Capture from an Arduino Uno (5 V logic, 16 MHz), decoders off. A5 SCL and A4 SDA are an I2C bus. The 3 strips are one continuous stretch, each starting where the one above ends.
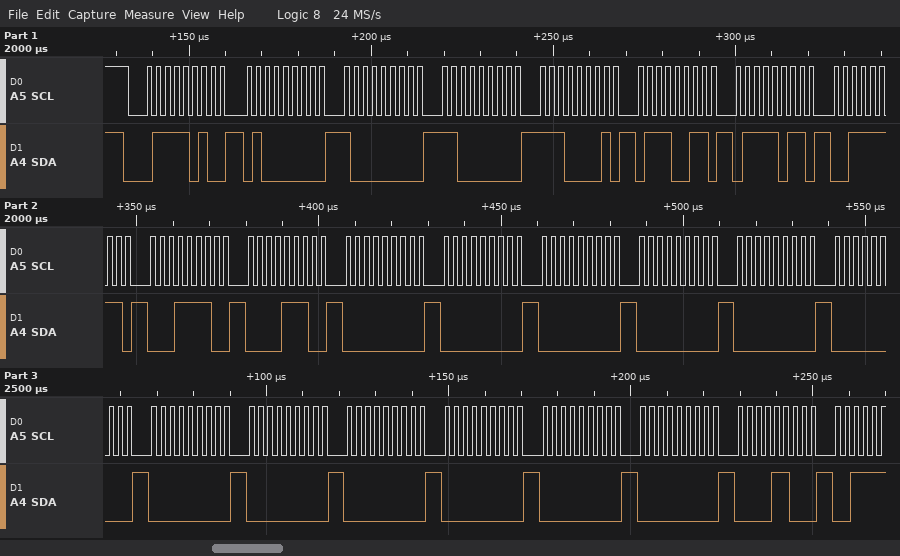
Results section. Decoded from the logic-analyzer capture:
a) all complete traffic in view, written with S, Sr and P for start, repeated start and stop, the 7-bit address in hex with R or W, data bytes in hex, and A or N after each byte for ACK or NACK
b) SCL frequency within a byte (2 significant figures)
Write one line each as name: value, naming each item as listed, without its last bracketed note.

all complete traffic in view, written with S, Sr and P for start, repeated start and stop, the 7-bit address in hex with R or W, data bytes in hex, and A or N after each byte for ACK or NACK: S 3DW A 40 A 80 A C0 A E1 A 73 A 7B A 3F A 1E A 0E A 00 A 00 A 00 A 00 A 00 A 00 A 00 A 00 A 00 A 00 A 00 A 00 A 0C A
SCL frequency within a byte: 400 kHz
